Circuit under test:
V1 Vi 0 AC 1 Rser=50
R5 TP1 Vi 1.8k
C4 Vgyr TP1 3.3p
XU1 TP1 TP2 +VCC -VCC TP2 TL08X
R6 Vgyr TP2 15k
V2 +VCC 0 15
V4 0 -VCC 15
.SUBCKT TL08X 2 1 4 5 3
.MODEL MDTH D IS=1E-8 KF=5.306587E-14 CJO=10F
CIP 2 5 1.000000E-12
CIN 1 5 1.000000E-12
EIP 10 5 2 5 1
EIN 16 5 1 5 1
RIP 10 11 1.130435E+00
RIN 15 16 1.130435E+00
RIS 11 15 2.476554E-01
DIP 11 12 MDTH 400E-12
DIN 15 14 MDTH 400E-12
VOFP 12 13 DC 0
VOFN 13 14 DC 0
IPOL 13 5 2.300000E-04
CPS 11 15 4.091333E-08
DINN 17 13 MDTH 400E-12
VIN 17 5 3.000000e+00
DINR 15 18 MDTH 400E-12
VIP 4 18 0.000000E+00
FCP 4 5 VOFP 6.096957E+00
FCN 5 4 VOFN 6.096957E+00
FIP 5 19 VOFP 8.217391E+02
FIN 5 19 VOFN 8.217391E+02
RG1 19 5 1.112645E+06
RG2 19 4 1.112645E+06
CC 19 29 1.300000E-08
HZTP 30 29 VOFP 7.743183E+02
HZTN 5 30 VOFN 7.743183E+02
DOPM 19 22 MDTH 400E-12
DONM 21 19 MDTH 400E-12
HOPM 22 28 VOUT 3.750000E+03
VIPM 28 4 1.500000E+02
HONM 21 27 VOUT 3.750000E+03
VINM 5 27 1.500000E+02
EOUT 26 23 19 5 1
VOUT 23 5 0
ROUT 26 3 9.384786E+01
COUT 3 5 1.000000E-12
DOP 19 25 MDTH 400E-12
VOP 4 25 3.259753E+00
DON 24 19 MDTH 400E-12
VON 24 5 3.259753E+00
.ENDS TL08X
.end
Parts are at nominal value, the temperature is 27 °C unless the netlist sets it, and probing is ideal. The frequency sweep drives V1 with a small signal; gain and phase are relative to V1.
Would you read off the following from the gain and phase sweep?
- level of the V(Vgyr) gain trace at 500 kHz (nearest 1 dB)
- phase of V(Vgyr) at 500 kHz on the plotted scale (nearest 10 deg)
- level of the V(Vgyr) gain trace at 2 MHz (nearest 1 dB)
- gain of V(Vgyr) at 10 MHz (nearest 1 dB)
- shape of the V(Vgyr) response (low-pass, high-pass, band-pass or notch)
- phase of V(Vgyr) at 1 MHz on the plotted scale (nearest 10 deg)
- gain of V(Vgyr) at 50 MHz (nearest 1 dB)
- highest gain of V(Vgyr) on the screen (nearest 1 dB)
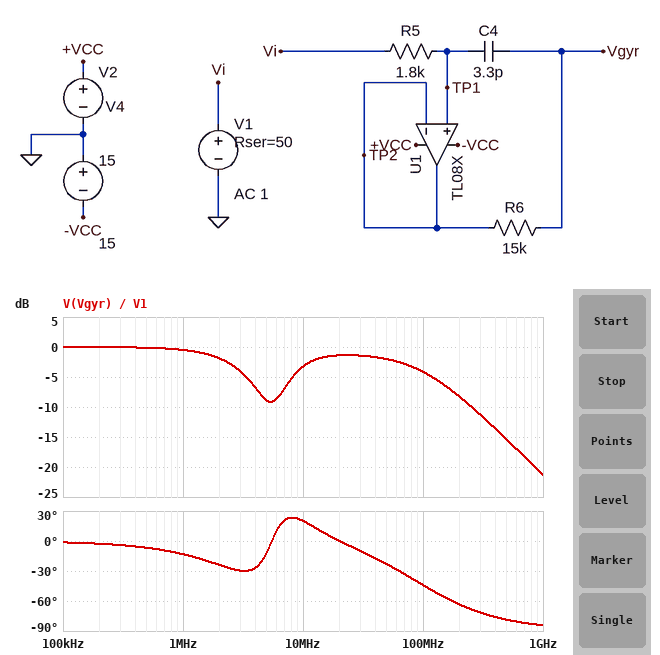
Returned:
0 dB
-10 deg
-2 dB
-3 dB
low-pass
-10 deg
-2 dB
0 dB
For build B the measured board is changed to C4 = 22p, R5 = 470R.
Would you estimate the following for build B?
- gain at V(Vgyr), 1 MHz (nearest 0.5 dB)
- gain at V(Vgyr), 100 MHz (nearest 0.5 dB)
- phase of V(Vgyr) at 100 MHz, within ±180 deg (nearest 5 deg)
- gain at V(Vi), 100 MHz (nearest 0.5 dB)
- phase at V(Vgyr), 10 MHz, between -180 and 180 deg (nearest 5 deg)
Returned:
-1.0 dB
-0.5 dB
-15 deg
0 dB
0 deg
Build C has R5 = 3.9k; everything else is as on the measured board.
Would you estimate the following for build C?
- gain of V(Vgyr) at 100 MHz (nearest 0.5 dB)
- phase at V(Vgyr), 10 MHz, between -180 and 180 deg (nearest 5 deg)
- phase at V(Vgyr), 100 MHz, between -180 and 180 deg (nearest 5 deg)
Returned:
-9.0 dB
10 deg
-60 deg
